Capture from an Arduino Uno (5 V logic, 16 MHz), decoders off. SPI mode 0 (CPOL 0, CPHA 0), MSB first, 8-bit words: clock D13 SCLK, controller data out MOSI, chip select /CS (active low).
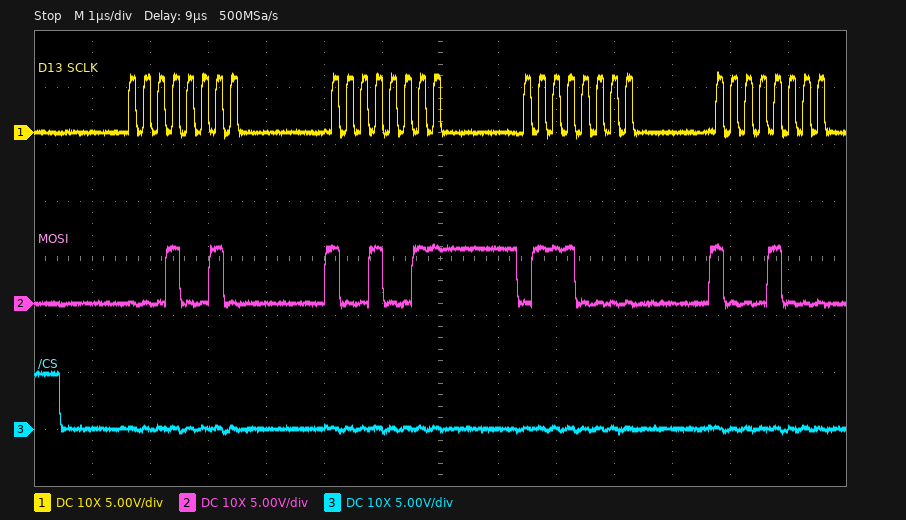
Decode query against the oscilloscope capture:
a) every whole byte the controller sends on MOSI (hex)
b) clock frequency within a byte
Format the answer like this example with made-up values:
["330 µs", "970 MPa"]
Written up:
["0x12 0x93 0x70 0x88", "4 MHz"]
